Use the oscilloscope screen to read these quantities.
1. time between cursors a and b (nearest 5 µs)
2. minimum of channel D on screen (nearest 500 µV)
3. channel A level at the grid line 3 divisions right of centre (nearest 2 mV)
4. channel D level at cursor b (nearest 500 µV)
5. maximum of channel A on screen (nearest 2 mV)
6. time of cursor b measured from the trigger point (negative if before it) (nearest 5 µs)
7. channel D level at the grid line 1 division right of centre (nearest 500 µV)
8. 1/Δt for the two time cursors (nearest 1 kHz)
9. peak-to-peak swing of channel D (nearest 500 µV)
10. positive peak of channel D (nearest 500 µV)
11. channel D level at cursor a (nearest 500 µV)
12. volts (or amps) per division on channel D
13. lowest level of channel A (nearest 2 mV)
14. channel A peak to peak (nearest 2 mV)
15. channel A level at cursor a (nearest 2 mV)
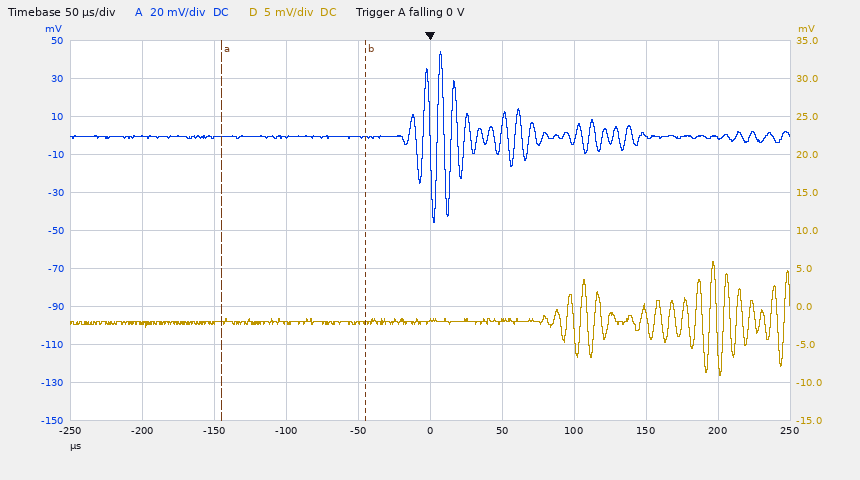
100 µs
-9.0 mV
0 mV
-2.0 mV
44 mV
-45 µs
-2.0 mV
10 kHz
15.0 mV
6.0 mV
-2.0 mV
5 mV
-46 mV
90 mV
0 mV
